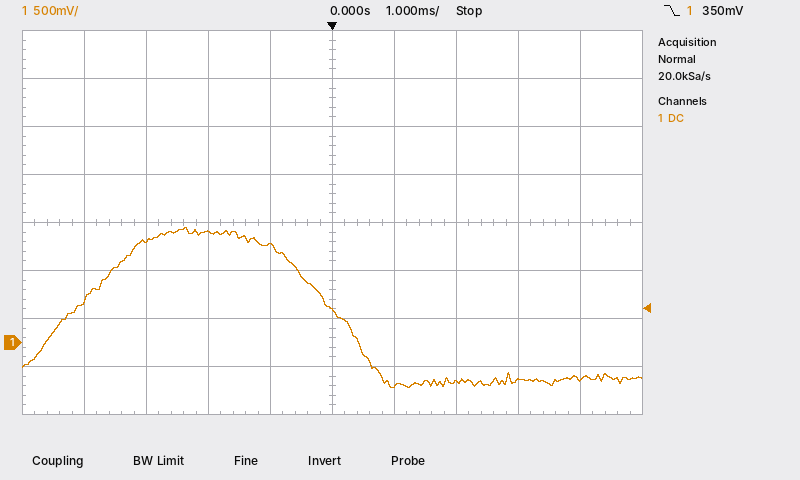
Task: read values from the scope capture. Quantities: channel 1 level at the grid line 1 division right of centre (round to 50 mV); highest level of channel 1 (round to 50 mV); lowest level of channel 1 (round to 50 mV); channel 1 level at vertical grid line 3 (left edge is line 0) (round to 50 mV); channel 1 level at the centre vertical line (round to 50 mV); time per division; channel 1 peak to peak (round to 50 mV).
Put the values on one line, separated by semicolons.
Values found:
-450 mV; 1.20 V; -450 mV; 1.15 V; 350 mV; 1 ms; 1.65 V
